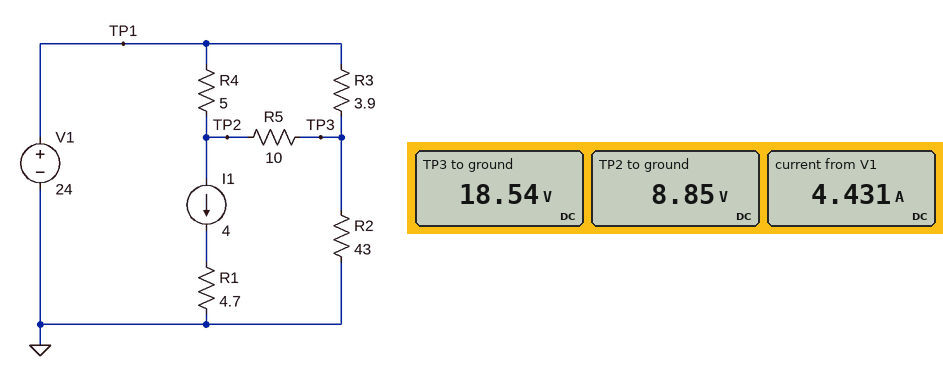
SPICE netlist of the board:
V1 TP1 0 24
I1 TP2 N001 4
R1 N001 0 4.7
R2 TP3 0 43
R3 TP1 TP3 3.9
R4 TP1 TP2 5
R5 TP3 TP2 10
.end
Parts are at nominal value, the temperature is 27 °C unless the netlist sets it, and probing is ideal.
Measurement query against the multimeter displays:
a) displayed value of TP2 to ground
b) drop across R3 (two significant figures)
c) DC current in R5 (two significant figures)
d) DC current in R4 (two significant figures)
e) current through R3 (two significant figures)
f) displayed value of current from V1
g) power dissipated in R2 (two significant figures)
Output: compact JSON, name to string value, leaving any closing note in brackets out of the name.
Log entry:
{"displayed value of TP2 to ground": "8.85 V", "drop across R3": "5.5 V", "DC current in R5": "970 mA", "DC current in R4": "3.0 A", "current through R3": "1.4 A", "displayed value of current from V1": "4.431 A", "power dissipated in R2": "8.0 W"}
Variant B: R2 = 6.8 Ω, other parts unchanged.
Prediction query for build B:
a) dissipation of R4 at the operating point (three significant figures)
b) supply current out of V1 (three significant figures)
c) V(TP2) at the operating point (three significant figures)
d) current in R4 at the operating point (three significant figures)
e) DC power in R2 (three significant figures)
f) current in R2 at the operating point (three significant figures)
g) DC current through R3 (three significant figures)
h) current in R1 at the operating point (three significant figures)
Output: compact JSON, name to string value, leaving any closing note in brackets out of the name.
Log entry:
{"dissipation of R4 at the operating point": "56.3 W", "supply current out of V1": "6.01 A", "V(TP2) at the operating point": "7.22 V", "current in R4 at the operating point": "3.36 A", "DC power in R2": "27.4 W", "current in R2 at the operating point": "2.01 A", "DC current through R3": "2.65 A", "current in R1 at the operating point": "4.00 A"}
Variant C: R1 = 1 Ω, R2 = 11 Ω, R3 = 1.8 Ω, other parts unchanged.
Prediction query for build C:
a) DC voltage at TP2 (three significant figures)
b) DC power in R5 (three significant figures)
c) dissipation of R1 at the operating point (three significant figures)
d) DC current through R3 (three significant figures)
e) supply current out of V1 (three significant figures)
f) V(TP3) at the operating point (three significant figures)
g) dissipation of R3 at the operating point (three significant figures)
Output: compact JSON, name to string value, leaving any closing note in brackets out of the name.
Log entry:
{"DC voltage at TP2": "9.02 V", "DC power in R5": "10.1 W", "dissipation of R1 at the operating point": "16.0 W", "DC current through R3": "2.74 A", "supply current out of V1": "5.73 A", "V(TP3) at the operating point": "19.1 V", "dissipation of R3 at the operating point": "13.5 W"}
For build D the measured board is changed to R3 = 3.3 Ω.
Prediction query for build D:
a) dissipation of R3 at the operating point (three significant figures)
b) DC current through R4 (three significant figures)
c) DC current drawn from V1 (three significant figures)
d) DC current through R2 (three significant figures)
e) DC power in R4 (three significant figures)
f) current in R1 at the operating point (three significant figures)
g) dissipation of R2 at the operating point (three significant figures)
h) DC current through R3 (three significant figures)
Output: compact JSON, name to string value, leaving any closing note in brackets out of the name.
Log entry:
{"dissipation of R3 at the operating point": "7.02 W", "DC current through R4": "2.99 A", "DC current drawn from V1": "4.45 A", "DC current through R2": "446 mA", "DC power in R4": "44.6 W", "current in R1 at the operating point": "4.00 A", "dissipation of R2 at the operating point": "8.56 W", "DC current through R3": "1.46 A"}
